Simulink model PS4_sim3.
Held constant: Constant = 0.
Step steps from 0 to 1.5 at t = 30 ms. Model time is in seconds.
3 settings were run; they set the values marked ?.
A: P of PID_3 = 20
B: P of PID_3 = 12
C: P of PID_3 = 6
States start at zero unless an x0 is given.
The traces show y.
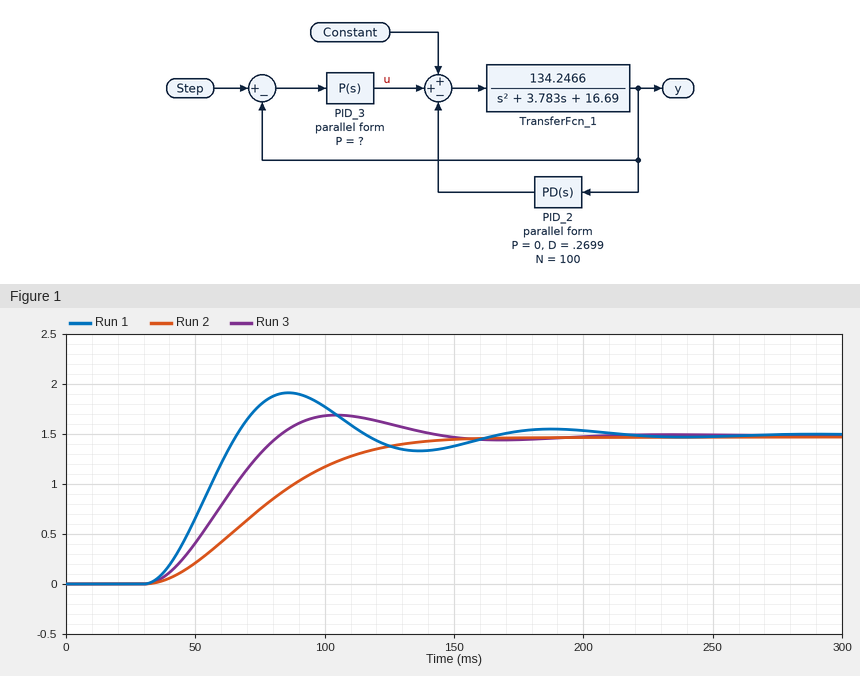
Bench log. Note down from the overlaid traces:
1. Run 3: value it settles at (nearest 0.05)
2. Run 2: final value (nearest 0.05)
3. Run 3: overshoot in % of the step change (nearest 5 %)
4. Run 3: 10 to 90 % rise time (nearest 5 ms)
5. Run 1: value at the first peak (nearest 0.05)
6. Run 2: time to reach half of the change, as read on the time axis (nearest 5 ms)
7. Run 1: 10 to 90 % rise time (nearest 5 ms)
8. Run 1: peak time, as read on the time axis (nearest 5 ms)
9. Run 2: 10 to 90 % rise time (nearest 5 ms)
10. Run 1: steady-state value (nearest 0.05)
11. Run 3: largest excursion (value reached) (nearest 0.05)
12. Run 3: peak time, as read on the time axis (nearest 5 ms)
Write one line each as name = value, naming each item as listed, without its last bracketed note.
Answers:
Run 3: value it settles at = 1.50
Run 2: final value = 1.45
Run 3: overshoot in % of the step change = 15 %
Run 3: 10 to 90 % rise time = 35 ms
Run 1: value at the first peak = 1.90
Run 2: time to reach half of the change, as read on the time axis = 75 ms
Run 1: 10 to 90 % rise time = 25 ms
Run 1: peak time, as read on the time axis = 85 ms
Run 2: 10 to 90 % rise time = 70 ms
Run 1: steady-state value = 1.50
Run 3: largest excursion (value reached) = 1.70
Run 3: peak time, as read on the time axis = 105 ms
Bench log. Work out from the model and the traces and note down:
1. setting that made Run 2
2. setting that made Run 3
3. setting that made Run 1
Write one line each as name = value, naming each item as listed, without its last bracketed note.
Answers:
setting that made Run 2 = C
setting that made Run 3 = B
setting that made Run 1 = A
